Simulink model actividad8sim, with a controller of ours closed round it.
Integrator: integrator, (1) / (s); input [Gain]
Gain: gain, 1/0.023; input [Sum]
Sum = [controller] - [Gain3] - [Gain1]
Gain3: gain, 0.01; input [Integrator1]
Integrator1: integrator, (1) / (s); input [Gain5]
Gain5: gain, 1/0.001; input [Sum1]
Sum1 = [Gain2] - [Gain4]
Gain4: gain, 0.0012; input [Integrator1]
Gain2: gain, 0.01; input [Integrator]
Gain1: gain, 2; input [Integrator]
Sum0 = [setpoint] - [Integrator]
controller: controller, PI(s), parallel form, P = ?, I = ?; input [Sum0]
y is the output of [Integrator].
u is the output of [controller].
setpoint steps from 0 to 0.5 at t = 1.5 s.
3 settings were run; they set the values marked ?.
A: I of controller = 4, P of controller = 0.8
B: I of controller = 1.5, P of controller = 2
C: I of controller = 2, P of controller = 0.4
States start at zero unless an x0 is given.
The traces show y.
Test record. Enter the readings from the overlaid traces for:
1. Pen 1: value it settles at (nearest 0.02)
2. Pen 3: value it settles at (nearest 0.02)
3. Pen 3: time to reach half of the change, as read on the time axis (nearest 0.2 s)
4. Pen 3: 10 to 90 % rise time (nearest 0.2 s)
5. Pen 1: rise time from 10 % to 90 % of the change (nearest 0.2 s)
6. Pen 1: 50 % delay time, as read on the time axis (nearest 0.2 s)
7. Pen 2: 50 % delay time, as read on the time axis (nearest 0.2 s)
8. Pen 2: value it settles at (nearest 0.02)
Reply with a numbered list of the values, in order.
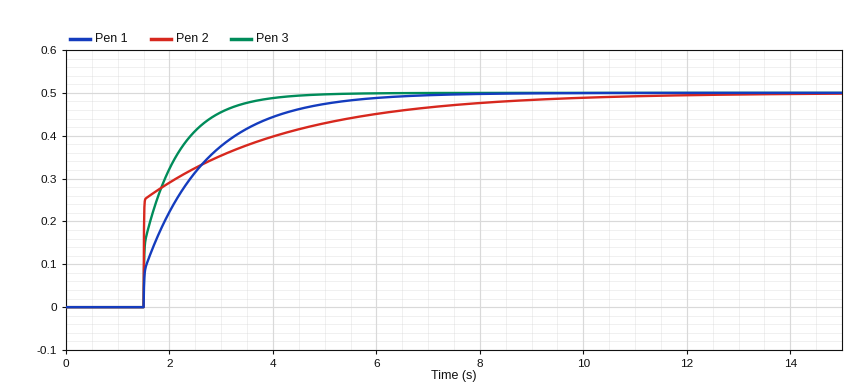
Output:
1. 0.50
2. 0.50
3. 1.8 s
4. 1.4 s
5. 2.6 s
6. 2.2 s
7. 1.6 s
8. 0.50
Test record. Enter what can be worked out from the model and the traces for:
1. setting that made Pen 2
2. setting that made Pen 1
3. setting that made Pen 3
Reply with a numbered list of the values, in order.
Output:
1. B
2. C
3. A
